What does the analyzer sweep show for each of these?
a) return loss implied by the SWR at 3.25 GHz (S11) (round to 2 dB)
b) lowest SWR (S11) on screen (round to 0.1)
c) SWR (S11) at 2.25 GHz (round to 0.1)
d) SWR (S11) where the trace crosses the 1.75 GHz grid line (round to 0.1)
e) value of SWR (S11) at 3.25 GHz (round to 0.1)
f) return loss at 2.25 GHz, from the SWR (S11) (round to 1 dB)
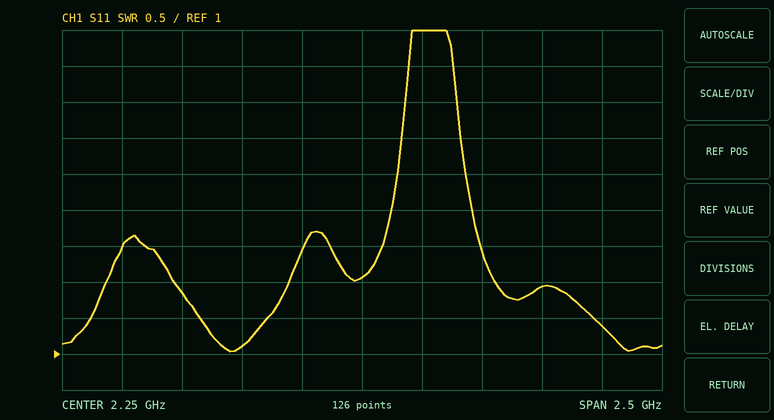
16 dB
1.0
2.1
1.1
1.4
9 dB
